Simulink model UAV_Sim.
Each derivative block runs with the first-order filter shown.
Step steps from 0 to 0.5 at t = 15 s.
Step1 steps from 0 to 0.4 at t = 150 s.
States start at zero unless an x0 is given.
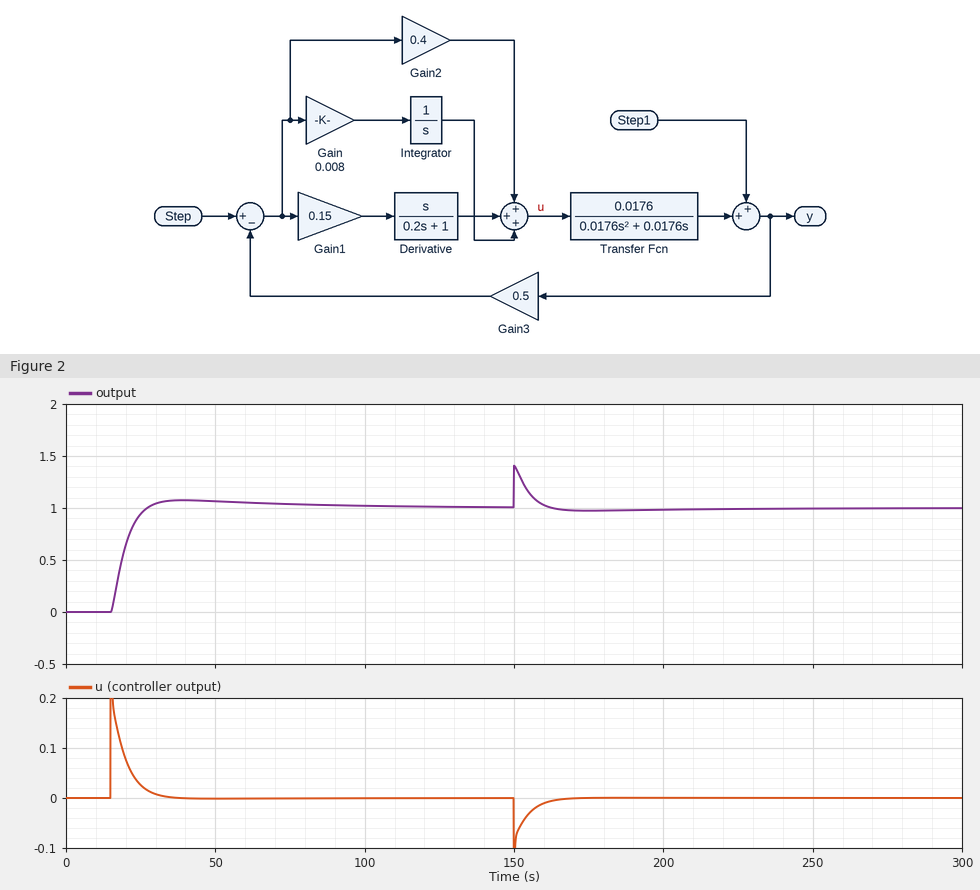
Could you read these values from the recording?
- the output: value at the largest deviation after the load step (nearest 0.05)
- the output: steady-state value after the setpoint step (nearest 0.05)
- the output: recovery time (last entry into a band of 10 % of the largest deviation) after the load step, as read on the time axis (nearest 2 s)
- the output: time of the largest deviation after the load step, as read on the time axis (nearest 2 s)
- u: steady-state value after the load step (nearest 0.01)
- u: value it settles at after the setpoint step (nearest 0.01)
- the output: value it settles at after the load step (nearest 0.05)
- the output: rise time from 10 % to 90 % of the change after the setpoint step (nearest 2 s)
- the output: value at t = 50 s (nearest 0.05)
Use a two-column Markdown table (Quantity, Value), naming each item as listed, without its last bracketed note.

| Quantity | Value |
|---|---|
| the output: value at the largest deviation after the load step | 1.40 |
| the output: steady-state value after the setpoint step | 1.00 |
| the output: recovery time (last entry into a band of 10 % of the largest deviation) after the load step, as read on the time axis | 160 s |
| the output: time of the largest deviation after the load step, as read on the time axis | 150 s |
| u: steady-state value after the load step | 0.00 |
| u: value it settles at after the setpoint step | 0.00 |
| the output: value it settles at after the load step | 1.00 |
| the output: rise time from 10 % to 90 % of the change after the setpoint step | 8 s |
| the output: value at t = 50 s | 1.05 |
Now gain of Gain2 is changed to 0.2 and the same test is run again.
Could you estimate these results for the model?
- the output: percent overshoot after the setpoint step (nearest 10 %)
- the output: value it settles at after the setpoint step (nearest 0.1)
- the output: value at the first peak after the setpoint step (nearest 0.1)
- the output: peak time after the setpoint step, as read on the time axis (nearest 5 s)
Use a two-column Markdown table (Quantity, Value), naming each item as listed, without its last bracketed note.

| Quantity | Value |
|---|---|
| the output: percent overshoot after the setpoint step | 20 % |
| the output: value it settles at after the setpoint step | 1.0 |
| the output: value at the first peak after the setpoint step | 1.2 |
| the output: peak time after the setpoint step, as read on the time axis | 50 s |
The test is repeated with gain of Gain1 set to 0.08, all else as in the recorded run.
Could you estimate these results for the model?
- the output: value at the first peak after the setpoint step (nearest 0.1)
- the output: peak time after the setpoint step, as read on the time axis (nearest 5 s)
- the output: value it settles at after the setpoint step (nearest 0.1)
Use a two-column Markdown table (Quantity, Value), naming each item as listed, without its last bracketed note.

| Quantity | Value |
|---|---|
| the output: value at the first peak after the setpoint step | 1.1 |
| the output: peak time after the setpoint step, as read on the time axis | 40 s |
| the output: value it settles at after the setpoint step | 1.0 |
